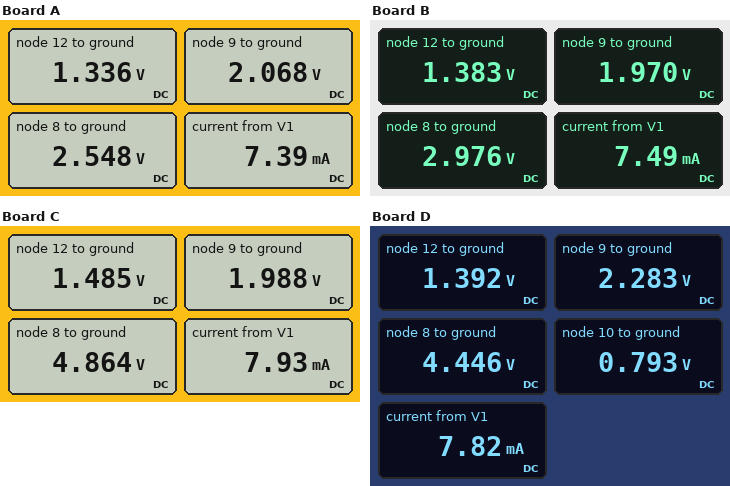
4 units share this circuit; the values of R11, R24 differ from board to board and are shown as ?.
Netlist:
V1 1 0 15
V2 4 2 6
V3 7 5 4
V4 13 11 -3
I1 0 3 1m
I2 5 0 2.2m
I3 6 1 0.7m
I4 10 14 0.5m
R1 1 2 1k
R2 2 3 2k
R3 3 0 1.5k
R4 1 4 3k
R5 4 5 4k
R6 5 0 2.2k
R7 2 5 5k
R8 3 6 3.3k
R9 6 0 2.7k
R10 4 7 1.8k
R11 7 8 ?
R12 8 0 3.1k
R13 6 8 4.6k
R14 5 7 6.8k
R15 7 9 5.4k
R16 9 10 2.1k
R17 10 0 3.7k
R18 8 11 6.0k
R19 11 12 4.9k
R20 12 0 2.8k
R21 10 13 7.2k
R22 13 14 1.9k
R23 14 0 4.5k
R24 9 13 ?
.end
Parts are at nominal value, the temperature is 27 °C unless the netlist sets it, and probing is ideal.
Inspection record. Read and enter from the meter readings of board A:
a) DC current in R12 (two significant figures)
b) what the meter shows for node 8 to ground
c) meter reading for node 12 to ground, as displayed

820 µA
2.548 V
1.336 V
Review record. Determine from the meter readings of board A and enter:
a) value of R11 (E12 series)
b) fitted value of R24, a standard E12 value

5.6 kΩ
3.3 kΩ
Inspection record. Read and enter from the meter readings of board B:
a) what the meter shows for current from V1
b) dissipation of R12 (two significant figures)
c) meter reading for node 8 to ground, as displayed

7.49 mA
2.9 mW
2.976 V
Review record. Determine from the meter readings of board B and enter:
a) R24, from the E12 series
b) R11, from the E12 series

2.7 kΩ
3.9 kΩ
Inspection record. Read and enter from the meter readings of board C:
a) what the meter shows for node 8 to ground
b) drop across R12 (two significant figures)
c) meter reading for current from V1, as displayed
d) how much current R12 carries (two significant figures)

4.864 V
4.9 V
7.93 mA
1.6 mA
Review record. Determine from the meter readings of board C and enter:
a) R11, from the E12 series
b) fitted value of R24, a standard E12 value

820 Ω
3.3 kΩ
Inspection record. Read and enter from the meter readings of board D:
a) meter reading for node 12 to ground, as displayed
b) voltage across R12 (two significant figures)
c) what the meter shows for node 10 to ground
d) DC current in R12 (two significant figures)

1.392 V
4.4 V
0.793 V
1.4 mA
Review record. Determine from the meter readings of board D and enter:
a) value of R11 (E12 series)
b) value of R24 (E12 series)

1.2 kΩ
8.2 kΩ
